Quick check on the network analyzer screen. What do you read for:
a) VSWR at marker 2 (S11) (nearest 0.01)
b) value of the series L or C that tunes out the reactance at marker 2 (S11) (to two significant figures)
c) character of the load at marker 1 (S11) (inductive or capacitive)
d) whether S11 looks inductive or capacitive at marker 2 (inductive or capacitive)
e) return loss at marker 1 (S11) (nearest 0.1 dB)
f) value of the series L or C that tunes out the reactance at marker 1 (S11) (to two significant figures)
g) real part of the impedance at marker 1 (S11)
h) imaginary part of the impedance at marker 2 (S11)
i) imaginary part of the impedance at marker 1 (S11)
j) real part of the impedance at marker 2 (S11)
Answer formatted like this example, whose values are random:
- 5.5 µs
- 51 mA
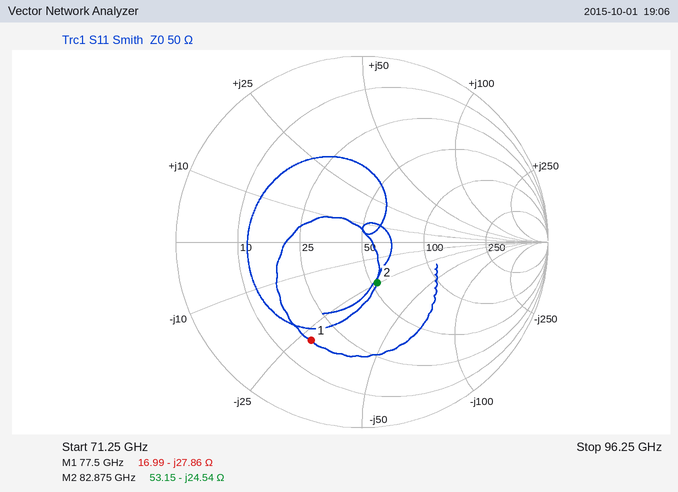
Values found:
- 1.61
- 47 pH
- capacitive
- capacitive
- 4.5 dB
- 57 pH
- 16.99 Ω
- -24.54 Ω
- -27.86 Ω
- 53.15 Ω
